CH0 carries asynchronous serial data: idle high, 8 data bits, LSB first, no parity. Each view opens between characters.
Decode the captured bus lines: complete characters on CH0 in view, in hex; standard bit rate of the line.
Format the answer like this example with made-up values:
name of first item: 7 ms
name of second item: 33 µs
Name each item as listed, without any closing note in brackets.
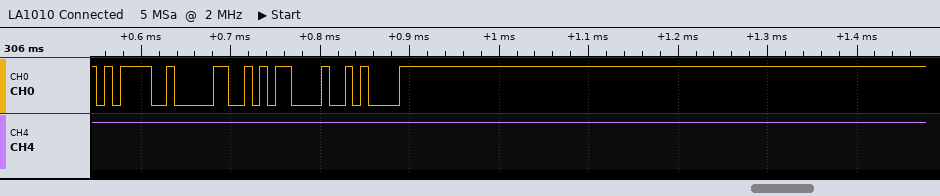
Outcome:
complete characters on CH0 in view, in hex: 3D, 30, 0D, 0A
standard bit rate of the line: 115200 baud
